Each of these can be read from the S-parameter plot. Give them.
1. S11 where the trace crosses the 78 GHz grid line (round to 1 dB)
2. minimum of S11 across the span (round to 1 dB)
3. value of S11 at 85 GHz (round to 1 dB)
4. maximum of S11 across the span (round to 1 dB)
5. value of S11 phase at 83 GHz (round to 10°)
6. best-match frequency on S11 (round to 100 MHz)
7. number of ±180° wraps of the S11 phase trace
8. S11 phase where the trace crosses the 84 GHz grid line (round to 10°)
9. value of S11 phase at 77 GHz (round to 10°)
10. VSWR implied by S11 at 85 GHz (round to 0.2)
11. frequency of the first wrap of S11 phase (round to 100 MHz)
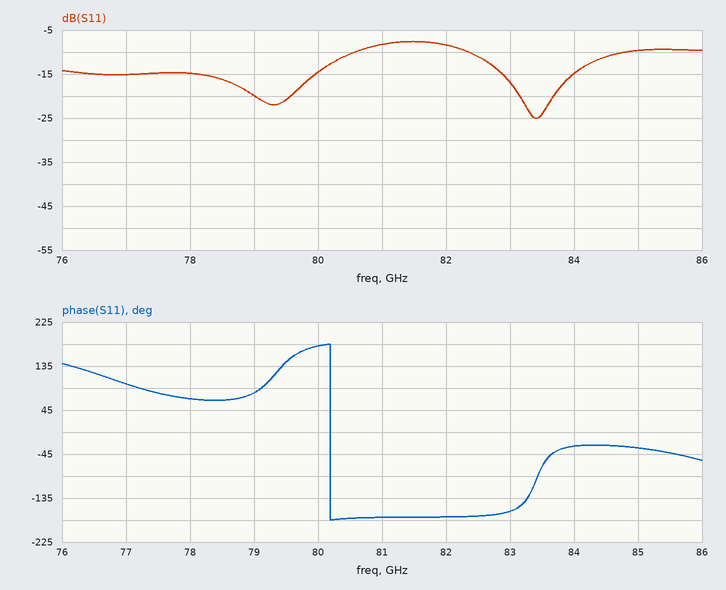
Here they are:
-15 dB
-25 dB
-10 dB
-8 dB
-160°
83.4 GHz
1
-30°
100°
2.0
80.2 GHz
